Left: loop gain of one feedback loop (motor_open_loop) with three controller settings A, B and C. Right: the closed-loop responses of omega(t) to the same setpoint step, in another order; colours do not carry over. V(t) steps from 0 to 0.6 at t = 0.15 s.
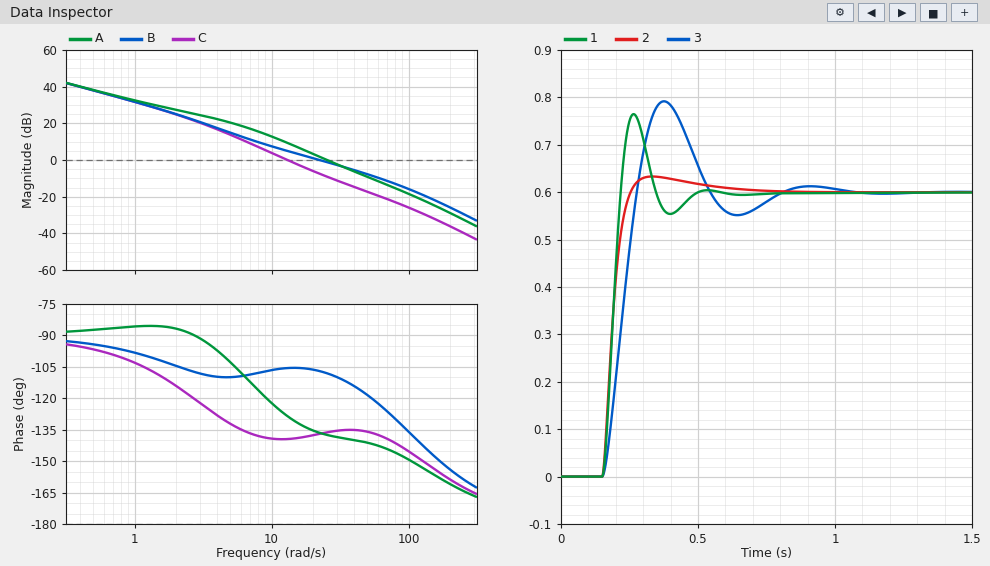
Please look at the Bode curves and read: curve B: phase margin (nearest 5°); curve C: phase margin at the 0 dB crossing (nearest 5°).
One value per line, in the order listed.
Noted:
75°
40°
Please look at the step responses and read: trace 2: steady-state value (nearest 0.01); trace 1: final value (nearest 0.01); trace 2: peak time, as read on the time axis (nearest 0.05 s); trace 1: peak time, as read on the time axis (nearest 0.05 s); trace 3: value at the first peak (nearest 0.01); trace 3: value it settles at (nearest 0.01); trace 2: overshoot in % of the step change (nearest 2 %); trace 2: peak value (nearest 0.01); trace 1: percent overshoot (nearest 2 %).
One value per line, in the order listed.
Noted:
0.60
0.60
0.35 s
0.25 s
0.79
0.60
6 %
0.63
28 %
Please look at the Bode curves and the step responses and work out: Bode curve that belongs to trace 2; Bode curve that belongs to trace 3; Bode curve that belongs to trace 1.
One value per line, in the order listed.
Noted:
B
C
A
